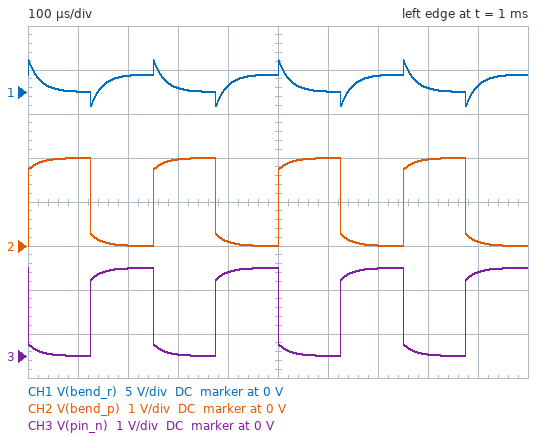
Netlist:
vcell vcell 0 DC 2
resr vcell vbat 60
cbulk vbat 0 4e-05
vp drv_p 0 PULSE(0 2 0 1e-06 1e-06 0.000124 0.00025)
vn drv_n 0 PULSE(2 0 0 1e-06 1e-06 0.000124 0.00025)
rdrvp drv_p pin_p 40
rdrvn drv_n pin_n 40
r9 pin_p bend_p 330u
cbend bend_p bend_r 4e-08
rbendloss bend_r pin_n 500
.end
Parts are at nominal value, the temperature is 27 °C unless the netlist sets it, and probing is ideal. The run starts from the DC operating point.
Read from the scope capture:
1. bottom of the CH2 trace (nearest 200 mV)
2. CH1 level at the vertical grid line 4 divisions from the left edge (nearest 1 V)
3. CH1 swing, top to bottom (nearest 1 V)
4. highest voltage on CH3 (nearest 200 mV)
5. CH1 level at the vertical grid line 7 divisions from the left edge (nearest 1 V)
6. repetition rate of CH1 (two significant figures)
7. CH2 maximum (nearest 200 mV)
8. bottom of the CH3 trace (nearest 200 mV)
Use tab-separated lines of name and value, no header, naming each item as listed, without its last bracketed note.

bottom of the CH2 trace	0 V
CH1 level at the vertical grid line 4 divisions from the left edge	1 V
CH1 swing, top to bottom	5 V
highest voltage on CH3	2.0 V
CH1 level at the vertical grid line 7 divisions from the left edge	2 V
repetition rate of CH1	4.0 kHz
CH2 maximum	2.0 V
bottom of the CH3 trace	0 V
